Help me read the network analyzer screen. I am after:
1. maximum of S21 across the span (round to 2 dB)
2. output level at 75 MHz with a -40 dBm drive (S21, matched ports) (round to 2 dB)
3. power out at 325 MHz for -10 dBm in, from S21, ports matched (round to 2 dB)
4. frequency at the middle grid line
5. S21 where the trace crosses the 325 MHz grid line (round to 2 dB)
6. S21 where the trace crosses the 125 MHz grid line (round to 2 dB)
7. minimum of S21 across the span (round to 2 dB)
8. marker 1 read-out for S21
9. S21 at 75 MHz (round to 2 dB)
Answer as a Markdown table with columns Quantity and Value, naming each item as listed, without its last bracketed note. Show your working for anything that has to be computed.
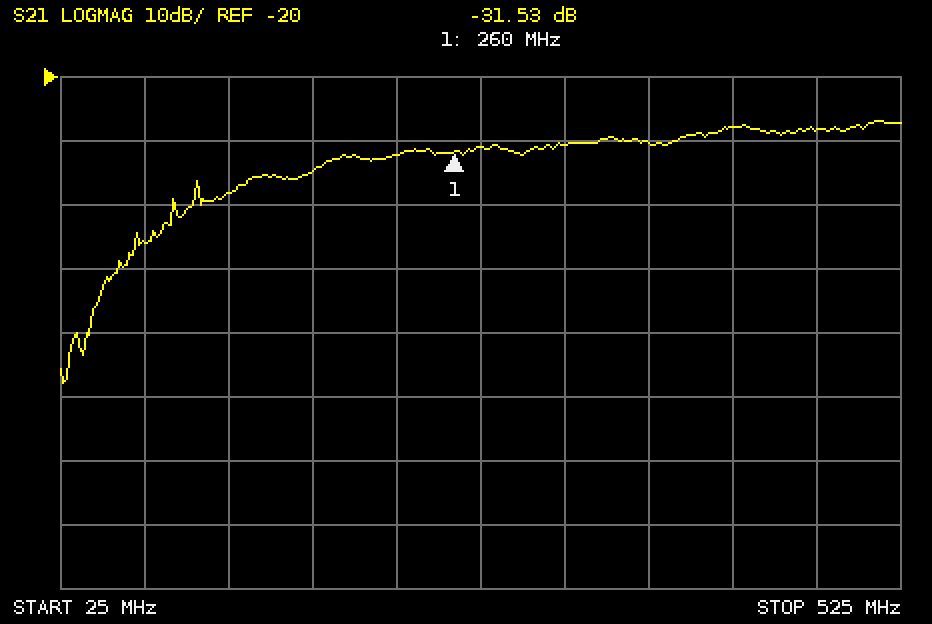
| Quantity | Value |
|---|---|
| maximum of S21 across the span | -26 dB |
| output level at 75 MHz with a -40 dBm drive (S21, matched ports) | -40 dBm + (-46 dB) = -86 dBm |
| power out at 325 MHz for -10 dBm in, from S21, ports matched | -10 dBm + (-30 dB) = -40 dBm |
| frequency at the middle grid line | 275 MHz |
| S21 where the trace crosses the 325 MHz grid line | -30 dB |
| S21 where the trace crosses the 125 MHz grid line | -38 dB |
| minimum of S21 across the span | -68 dB |
| marker 1 read-out for S21 | -31.53 dB |
| S21 at 75 MHz | -46 dB |
